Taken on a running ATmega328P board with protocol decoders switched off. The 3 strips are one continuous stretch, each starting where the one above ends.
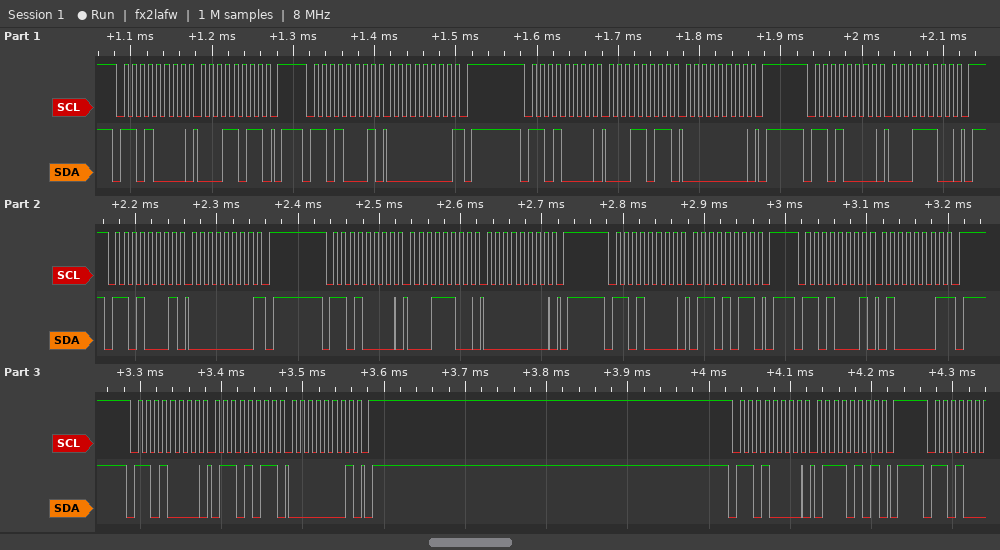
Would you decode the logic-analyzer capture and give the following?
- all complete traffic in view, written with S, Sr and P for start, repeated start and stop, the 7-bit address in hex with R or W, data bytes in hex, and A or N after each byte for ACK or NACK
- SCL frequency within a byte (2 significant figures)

S 68W A 1B A P S 68R A 00 N P S 68W A 1B A 00 A P S 68W A 1C A P S 68R A 00 N P S 68W A 1C A 00 A P S 68W A 6B A P S 68R A 41 N P S 68W A 6B A 01 A P S 68W A 75 A P
100 kHz
